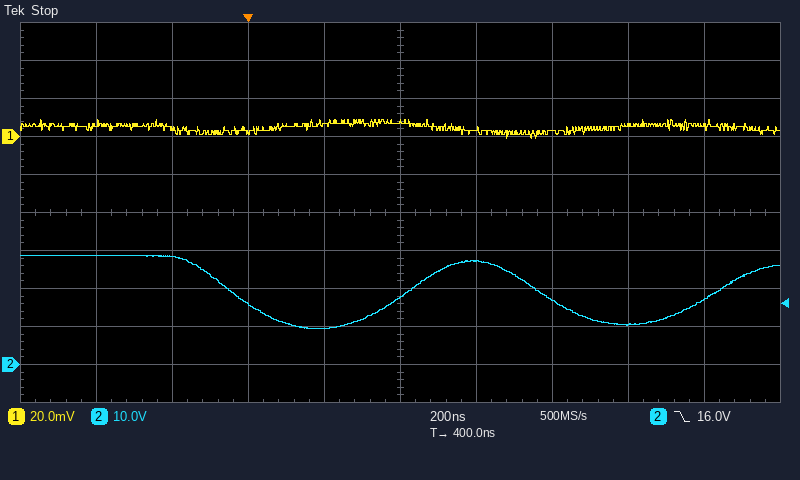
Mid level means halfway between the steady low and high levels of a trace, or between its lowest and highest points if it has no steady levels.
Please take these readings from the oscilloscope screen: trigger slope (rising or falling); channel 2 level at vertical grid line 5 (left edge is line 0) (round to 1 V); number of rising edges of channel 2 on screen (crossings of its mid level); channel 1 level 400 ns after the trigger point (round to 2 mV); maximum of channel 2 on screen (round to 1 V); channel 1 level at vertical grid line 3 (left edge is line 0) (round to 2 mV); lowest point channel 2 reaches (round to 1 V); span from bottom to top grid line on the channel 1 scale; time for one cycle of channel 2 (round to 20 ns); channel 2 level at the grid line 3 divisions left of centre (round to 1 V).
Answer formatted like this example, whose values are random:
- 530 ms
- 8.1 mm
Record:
- falling
- 18 V
- 2
- 8 mV
- 29 V
- 2 mV
- 9 V
- 200 mV
- 820 ns
- 28 V
